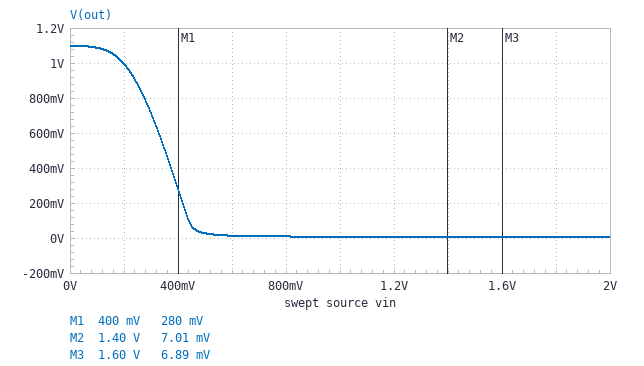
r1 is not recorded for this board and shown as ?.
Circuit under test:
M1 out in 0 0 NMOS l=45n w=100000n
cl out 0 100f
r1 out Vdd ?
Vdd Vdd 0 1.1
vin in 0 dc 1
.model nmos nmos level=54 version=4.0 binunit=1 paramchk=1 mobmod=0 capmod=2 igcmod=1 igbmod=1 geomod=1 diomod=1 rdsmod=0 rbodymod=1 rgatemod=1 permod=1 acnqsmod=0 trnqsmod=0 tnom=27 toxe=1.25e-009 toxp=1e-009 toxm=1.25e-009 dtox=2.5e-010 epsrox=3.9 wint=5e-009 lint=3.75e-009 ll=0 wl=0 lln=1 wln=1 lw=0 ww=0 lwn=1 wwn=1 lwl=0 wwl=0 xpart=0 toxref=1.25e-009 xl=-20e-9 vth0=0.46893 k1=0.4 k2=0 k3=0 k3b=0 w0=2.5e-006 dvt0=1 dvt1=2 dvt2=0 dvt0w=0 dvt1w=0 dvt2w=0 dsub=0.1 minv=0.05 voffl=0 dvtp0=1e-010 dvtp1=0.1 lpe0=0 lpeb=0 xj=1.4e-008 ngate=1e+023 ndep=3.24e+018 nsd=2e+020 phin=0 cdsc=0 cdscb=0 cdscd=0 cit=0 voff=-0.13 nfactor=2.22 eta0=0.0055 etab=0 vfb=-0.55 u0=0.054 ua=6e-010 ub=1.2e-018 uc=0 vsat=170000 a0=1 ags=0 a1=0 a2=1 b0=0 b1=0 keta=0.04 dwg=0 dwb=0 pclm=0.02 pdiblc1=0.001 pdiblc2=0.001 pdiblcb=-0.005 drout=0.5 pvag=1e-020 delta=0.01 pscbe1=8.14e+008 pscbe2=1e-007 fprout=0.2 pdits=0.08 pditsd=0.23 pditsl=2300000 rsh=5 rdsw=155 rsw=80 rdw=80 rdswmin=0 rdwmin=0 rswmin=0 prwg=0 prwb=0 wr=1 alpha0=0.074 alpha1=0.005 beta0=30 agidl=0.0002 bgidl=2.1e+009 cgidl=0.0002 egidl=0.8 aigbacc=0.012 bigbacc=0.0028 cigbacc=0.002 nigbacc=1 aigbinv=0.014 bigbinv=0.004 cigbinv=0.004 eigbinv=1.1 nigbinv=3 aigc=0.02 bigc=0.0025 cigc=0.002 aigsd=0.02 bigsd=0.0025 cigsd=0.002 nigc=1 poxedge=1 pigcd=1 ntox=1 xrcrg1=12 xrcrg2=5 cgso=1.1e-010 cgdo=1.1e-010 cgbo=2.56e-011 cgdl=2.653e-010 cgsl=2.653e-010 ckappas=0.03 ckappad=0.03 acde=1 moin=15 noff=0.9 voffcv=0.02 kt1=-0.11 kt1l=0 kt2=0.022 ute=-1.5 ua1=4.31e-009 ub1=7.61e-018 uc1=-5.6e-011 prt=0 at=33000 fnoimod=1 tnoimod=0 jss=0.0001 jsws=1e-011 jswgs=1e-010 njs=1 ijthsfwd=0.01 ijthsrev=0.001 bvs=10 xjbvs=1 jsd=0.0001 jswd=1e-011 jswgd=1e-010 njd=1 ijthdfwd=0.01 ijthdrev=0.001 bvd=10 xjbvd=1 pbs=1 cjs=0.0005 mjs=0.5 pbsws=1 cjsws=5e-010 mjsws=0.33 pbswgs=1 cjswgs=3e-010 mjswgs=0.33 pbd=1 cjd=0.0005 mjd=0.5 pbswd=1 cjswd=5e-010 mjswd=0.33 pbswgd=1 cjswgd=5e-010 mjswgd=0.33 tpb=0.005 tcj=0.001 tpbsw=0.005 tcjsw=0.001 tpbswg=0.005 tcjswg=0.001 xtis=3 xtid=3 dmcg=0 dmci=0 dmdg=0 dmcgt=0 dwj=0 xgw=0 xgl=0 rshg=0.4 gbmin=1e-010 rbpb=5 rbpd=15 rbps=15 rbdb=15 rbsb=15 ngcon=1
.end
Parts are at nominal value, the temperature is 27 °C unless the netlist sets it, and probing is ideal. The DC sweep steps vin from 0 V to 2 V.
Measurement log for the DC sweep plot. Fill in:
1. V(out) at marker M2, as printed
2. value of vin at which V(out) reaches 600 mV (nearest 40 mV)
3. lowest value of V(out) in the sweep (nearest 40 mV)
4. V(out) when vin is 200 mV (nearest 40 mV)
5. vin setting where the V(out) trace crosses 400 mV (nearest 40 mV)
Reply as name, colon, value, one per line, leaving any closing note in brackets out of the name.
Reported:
V(out) at marker M2, as printed: 7.01 mV
value of vin at which V(out) reaches 600 mV: 320 mV
lowest value of V(out) in the sweep: 0 V
V(out) when vin is 200 mV: 1.00 V
vin setting where the V(out) trace crosses 400 mV: 360 mV
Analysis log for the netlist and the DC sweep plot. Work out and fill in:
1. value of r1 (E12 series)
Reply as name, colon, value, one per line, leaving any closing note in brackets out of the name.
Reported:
value of r1: 330 Ω
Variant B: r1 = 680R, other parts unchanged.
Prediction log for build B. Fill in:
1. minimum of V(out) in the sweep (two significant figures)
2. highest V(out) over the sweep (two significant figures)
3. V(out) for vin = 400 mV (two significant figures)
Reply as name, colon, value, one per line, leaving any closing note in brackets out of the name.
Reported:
minimum of V(out) in the sweep: 3.3 mV
highest V(out) over the sweep: 1.1 V
V(out) for vin = 400 mV: 99 mV
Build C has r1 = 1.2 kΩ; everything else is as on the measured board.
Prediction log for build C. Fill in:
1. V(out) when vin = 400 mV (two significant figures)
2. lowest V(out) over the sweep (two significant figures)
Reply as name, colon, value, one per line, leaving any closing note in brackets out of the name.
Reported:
V(out) when vin = 400 mV: 33 mV
lowest V(out) over the sweep: 1.9 mV
